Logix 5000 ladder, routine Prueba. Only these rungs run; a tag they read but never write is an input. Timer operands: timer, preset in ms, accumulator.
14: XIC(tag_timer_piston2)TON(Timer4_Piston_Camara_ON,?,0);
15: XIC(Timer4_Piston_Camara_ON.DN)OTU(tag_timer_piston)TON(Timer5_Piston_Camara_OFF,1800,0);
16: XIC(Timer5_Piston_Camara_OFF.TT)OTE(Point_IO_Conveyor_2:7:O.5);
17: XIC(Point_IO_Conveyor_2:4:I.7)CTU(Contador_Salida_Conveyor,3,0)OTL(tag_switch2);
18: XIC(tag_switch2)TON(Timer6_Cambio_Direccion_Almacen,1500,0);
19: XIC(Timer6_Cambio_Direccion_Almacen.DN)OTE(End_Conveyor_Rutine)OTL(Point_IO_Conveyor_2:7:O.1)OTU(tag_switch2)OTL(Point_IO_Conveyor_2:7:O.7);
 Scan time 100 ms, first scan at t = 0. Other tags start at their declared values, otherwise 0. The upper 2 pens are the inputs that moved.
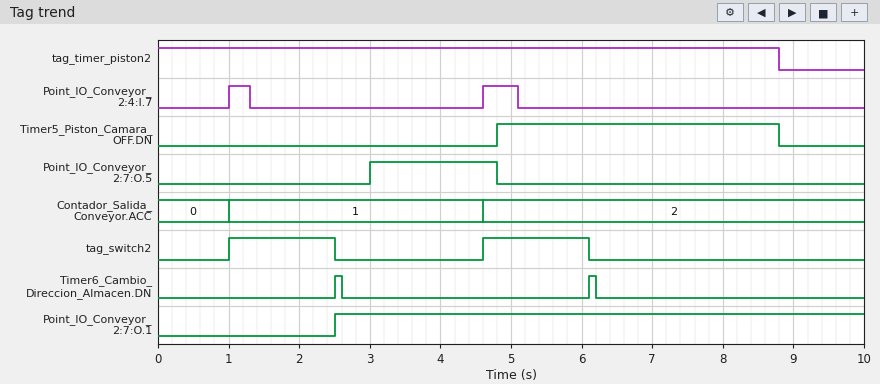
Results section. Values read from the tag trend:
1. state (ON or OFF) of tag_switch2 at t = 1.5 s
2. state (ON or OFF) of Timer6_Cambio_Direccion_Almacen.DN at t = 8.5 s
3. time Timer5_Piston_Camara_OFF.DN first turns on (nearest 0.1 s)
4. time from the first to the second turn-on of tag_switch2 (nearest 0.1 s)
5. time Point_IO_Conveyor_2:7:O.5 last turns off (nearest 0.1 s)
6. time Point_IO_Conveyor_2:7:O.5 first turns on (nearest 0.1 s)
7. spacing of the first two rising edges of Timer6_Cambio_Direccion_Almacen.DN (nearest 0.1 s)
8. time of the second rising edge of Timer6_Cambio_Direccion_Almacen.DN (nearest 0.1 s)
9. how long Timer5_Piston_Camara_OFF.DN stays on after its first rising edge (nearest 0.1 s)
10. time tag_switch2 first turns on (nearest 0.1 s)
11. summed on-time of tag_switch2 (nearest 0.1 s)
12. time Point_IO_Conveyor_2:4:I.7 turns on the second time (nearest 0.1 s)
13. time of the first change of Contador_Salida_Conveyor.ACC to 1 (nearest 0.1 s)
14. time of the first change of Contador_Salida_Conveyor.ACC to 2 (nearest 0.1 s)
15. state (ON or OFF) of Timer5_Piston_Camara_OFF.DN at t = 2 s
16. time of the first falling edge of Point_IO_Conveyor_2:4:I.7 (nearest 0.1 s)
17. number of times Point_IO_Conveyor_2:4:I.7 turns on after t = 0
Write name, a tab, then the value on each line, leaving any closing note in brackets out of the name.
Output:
state (ON or OFF) of tag_switch2 at t = 1.5 s	ON
state (ON or OFF) of Timer6_Cambio_Direccion_Almacen.DN at t = 8.5 s	OFF
time Timer5_Piston_Camara_OFF.DN first turns on	4.8 s
time from the first to the second turn-on of tag_switch2	3.6 s
time Point_IO_Conveyor_2:7:O.5 last turns off	4.8 s
time Point_IO_Conveyor_2:7:O.5 first turns on	3.0 s
spacing of the first two rising edges of Timer6_Cambio_Direccion_Almacen.DN	3.6 s
time of the second rising edge of Timer6_Cambio_Direccion_Almacen.DN	6.1 s
how long Timer5_Piston_Camara_OFF.DN stays on after its first rising edge	4.0 s
time tag_switch2 first turns on	1.0 s
summed on-time of tag_switch2	3.0 s
time Point_IO_Conveyor_2:4:I.7 turns on the second time	4.6 s
time of the first change of Contador_Salida_Conveyor.ACC to 1	1.0 s
time of the first change of Contador_Salida_Conveyor.ACC to 2	4.6 s
state (ON or OFF) of Timer5_Piston_Camara_OFF.DN at t = 2 s	OFF
time of the first falling edge of Point_IO_Conveyor_2:4:I.7	1.3 s
number of times Point_IO_Conveyor_2:4:I.7 turns on after t = 0	2
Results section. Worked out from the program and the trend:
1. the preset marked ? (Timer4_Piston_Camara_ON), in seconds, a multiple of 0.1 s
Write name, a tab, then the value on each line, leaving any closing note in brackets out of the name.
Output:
the preset marked ? (Timer4_Piston_Camara_ON), in seconds, a multiple of 0.1 s	3.0 s
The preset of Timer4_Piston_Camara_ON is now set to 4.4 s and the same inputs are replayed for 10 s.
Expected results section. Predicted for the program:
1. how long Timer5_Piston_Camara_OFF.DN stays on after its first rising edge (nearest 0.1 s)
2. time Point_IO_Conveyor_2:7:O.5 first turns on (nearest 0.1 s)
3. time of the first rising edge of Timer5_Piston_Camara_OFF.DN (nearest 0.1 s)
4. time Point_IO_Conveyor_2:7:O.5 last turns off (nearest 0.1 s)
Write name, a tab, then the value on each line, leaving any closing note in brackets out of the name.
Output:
how long Timer5_Piston_Camara_OFF.DN stays on after its first rising edge	2.6 s
time Point_IO_Conveyor_2:7:O.5 first turns on	4.4 s
time of the first rising edge of Timer5_Piston_Camara_OFF.DN	6.2 s
time Point_IO_Conveyor_2:7:O.5 last turns off	6.2 s
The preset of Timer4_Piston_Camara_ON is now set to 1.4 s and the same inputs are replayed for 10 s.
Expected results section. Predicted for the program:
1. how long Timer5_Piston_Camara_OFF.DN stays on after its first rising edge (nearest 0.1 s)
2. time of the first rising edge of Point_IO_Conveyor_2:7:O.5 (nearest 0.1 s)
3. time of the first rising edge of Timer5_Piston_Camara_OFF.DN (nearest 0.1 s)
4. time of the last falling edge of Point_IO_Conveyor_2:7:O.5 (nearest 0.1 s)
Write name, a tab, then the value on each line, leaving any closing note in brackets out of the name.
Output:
how long Timer5_Piston_Camara_OFF.DN stays on after its first rising edge	5.6 s
time of the first rising edge of Point_IO_Conveyor_2:7:O.5	1.4 s
time of the first rising edge of Timer5_Piston_Camara_OFF.DN	3.2 s
time of the last falling edge of Point_IO_Conveyor_2:7:O.5	3.2 s
